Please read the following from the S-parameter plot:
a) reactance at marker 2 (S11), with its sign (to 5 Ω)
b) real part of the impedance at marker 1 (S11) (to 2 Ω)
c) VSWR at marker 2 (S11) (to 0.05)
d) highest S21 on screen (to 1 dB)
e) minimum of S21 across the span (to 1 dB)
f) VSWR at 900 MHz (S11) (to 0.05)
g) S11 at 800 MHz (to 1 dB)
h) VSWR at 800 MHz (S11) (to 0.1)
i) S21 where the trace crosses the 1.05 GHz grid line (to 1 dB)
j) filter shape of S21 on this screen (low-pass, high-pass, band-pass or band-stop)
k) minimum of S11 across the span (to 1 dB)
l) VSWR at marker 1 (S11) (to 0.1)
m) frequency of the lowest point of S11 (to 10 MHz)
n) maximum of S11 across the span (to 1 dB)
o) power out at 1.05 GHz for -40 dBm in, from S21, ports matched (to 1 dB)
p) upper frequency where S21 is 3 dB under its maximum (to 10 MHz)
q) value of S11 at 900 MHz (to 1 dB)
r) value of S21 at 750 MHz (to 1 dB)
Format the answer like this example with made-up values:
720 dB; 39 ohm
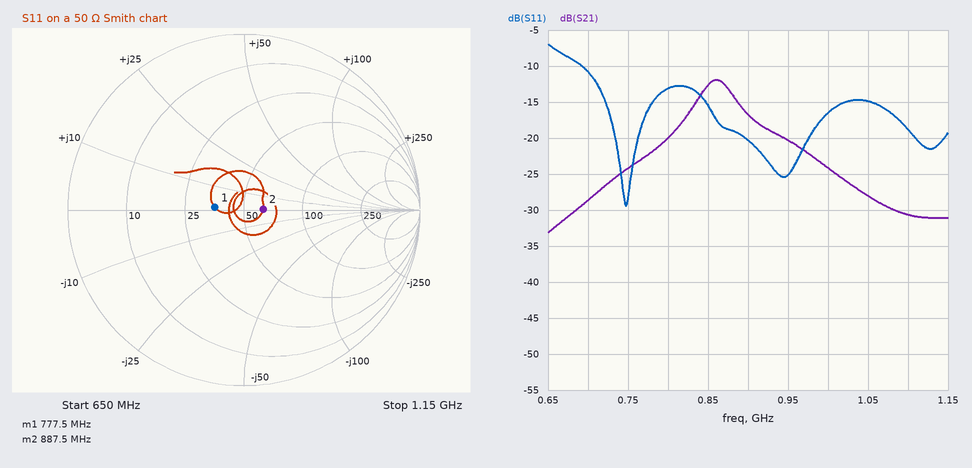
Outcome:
0 Ω; 36 Ω; 1.25; -12 dB; -33 dB; 1.20; -13 dB; 1.6; -28 dB; band-pass; -29 dB; 1.4; 750 MHz; -7 dB; -68 dBm; 890 MHz; -20 dB; -24 dB
